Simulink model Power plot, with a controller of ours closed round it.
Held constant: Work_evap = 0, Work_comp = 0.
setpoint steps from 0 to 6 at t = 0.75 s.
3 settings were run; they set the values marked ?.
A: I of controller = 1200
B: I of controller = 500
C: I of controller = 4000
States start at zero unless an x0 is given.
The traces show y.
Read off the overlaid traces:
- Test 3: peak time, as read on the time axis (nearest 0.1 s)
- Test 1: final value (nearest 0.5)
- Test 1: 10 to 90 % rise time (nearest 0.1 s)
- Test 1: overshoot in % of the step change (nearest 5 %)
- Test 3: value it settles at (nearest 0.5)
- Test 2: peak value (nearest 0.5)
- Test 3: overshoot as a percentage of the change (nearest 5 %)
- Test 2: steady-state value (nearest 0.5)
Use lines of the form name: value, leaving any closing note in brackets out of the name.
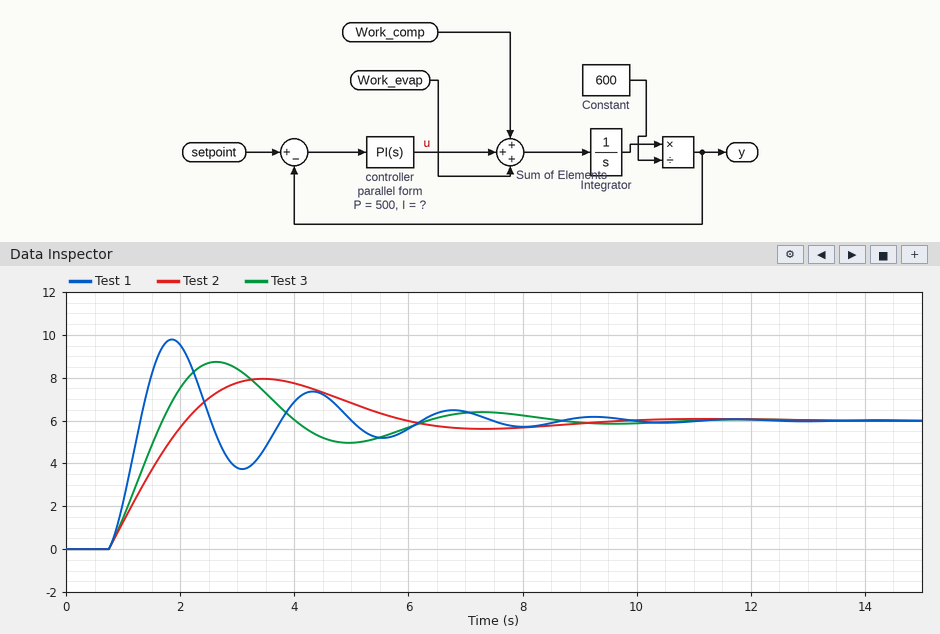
Test 3: peak time, as read on the time axis: 2.6 s
Test 1: final value: 6.0
Test 1: 10 to 90 % rise time: 0.4 s
Test 1: overshoot in % of the step change: 65 %
Test 3: value it settles at: 6.0
Test 2: peak value: 8.0
Test 3: overshoot as a percentage of the change: 45 %
Test 2: steady-state value: 6.0
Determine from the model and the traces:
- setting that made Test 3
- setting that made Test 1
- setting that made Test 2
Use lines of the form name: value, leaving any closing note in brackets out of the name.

setting that made Test 3: A
setting that made Test 1: C
setting that made Test 2: B
